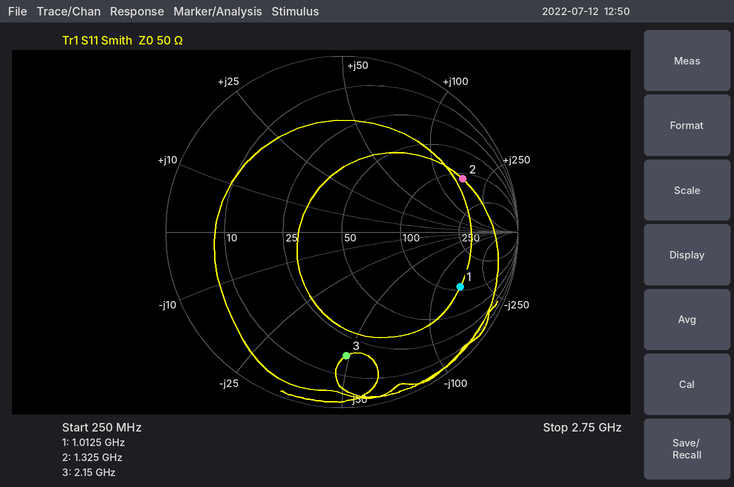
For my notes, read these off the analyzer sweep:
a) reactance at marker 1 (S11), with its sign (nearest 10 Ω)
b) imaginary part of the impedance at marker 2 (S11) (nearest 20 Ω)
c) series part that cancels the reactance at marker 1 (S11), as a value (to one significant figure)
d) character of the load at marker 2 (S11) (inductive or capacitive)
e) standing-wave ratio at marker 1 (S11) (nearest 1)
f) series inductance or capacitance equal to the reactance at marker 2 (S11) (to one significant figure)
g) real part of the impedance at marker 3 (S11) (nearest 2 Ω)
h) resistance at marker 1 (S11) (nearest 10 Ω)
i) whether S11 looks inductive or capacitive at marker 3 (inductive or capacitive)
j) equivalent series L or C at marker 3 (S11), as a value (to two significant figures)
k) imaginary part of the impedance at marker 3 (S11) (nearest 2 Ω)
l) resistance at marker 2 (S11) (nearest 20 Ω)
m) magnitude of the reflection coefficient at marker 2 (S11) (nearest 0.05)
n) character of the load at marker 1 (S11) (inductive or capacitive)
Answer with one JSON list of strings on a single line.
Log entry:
["-150 Ω", "+160 Ω", "20 nH", "inductive", "7", "20 nH", "18 Ω", "110 Ω", "capacitive", "1.5 pF", "-48 Ω", "120 Ω", "0.75", "capacitive"]
